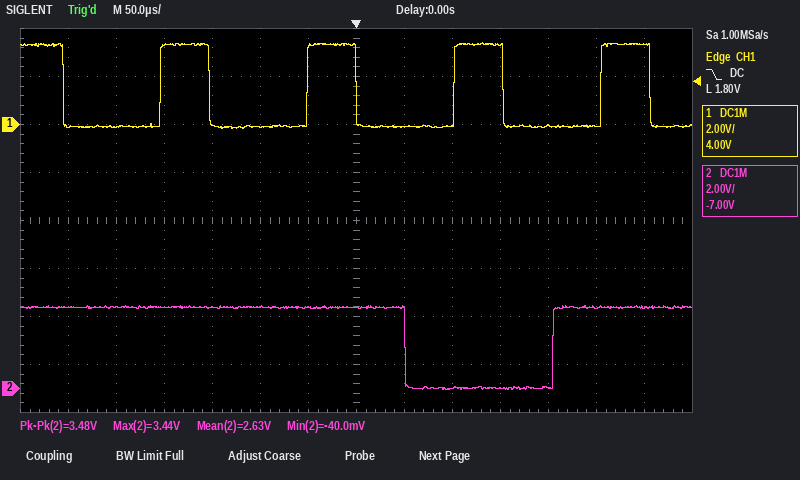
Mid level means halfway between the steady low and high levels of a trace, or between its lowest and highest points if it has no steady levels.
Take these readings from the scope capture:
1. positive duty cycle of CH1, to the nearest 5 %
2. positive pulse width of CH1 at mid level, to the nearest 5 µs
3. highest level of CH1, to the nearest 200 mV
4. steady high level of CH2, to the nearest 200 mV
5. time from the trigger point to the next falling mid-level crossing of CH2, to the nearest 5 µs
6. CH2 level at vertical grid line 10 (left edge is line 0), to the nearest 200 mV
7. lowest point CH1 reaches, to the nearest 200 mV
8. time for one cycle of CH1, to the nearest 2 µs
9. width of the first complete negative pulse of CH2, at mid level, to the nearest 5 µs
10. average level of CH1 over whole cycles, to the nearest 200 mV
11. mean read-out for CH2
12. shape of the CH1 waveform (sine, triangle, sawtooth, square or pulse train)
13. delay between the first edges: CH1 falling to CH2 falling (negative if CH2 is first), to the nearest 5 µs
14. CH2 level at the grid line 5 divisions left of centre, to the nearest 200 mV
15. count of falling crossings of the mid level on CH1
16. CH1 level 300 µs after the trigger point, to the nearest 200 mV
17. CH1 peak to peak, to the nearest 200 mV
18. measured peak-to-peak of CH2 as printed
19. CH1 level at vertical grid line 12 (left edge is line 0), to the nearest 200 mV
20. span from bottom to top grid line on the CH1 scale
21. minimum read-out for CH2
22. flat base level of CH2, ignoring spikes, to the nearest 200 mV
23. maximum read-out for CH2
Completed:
35 %
50 µs
3.4 V
3.4 V
50 µs
0.0 V
-200 mV
152 µs
155 µs
1.0 V
2.63 V
pulse train
+355 µs
3.4 V
5
3.4 V
3.6 V
3.48 V
0.0 V
16 V
-40.0 mV
0.0 V
3.44 V
